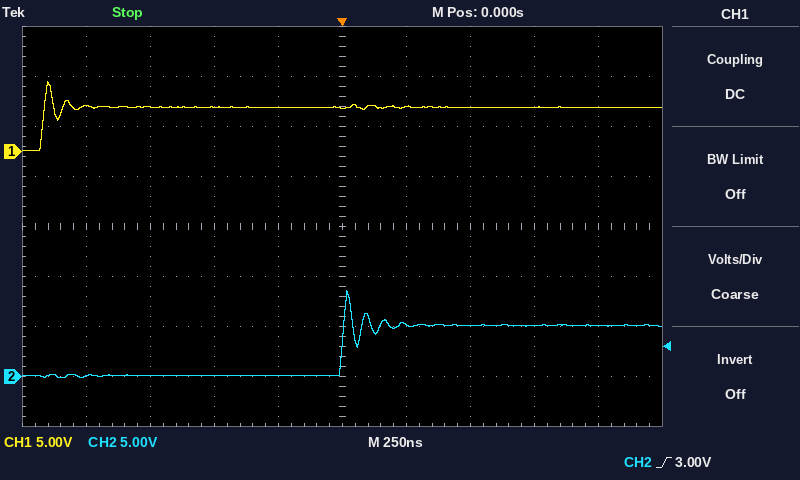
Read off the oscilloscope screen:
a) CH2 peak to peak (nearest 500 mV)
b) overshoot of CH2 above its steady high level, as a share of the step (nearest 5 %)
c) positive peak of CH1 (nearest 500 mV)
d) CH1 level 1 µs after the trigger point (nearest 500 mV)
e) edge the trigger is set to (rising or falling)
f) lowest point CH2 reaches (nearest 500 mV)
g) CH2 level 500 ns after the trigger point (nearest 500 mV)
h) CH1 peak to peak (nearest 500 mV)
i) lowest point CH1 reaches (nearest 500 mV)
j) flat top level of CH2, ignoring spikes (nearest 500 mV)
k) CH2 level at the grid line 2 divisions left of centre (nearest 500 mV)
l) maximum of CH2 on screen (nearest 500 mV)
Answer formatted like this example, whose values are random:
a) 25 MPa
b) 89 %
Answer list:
a) 8.5 V
b) 70 %
c) 7.0 V
d) 4.5 V
e) rising
f) 0.0 V
g) 5.0 V
h) 7.0 V
i) 0.0 V
j) 5.0 V
k) 0.0 V
l) 8.5 V
